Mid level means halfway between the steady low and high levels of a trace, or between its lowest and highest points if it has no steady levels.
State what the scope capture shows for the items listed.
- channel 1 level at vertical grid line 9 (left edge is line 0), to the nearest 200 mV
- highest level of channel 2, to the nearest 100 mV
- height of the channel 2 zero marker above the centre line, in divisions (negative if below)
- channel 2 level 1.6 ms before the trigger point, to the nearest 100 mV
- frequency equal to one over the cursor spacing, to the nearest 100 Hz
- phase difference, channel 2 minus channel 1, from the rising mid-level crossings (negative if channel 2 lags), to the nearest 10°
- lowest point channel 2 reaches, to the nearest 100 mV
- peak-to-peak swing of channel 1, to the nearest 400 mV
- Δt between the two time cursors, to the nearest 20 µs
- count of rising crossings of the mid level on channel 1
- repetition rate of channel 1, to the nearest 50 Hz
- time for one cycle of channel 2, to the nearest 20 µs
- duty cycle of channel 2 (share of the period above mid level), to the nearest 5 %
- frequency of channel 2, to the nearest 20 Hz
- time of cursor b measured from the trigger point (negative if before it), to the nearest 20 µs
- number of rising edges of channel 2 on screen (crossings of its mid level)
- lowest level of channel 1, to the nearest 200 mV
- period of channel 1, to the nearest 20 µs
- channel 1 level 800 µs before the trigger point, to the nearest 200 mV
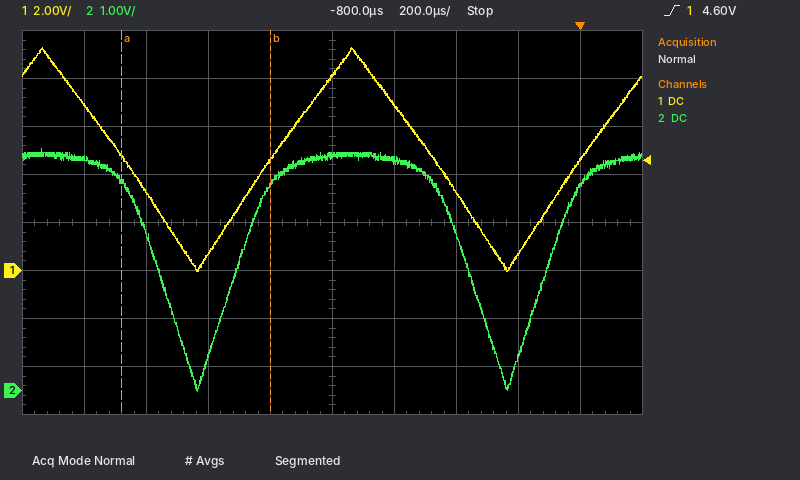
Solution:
4.6 V
5.0 V
-3.5 div
4.8 V
2.1 kHz
+40°
0.0 V
9.2 V
480 µs
2
1.00 kHz
1.00 ms
75 %
1.00 kHz
-1.00 ms
2
0.0 V
1.00 ms
8.2 V
